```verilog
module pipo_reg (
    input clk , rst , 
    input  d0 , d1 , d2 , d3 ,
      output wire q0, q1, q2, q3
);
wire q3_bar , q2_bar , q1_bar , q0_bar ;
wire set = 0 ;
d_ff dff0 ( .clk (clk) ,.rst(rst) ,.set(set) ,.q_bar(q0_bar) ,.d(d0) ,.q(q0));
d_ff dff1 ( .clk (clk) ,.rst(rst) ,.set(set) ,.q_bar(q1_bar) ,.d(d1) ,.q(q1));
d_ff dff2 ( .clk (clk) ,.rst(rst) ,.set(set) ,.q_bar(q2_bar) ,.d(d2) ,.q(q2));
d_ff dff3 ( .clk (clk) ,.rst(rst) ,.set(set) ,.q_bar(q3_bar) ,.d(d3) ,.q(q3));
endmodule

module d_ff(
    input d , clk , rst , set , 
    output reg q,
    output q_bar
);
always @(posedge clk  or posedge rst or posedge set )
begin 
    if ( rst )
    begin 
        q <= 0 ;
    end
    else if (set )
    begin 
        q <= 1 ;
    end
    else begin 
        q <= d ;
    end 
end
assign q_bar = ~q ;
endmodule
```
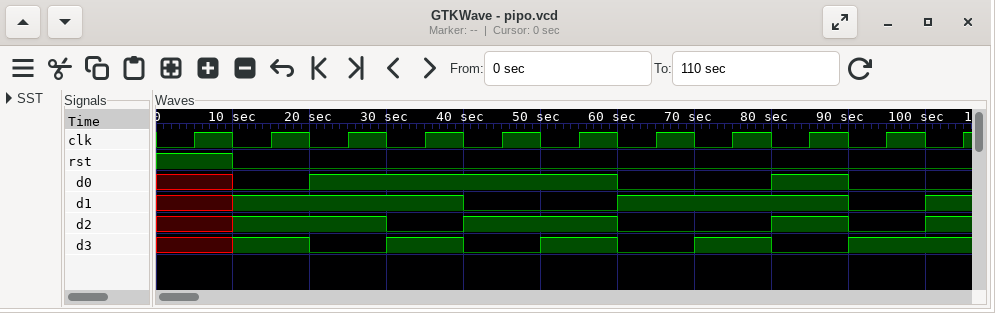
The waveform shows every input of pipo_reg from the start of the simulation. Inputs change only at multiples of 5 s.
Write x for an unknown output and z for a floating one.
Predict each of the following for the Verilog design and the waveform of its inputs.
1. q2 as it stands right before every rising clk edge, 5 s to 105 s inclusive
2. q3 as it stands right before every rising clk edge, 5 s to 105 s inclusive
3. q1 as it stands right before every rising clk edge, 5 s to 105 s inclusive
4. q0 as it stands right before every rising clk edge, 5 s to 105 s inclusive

0 0 1 1 0 1 1 0 0 1 0
0 0 1 0 1 0 1 0 1 0 1
0 0 1 1 1 0 0 1 1 1 0
0 0 0 1 1 1 1 0 0 1 0
